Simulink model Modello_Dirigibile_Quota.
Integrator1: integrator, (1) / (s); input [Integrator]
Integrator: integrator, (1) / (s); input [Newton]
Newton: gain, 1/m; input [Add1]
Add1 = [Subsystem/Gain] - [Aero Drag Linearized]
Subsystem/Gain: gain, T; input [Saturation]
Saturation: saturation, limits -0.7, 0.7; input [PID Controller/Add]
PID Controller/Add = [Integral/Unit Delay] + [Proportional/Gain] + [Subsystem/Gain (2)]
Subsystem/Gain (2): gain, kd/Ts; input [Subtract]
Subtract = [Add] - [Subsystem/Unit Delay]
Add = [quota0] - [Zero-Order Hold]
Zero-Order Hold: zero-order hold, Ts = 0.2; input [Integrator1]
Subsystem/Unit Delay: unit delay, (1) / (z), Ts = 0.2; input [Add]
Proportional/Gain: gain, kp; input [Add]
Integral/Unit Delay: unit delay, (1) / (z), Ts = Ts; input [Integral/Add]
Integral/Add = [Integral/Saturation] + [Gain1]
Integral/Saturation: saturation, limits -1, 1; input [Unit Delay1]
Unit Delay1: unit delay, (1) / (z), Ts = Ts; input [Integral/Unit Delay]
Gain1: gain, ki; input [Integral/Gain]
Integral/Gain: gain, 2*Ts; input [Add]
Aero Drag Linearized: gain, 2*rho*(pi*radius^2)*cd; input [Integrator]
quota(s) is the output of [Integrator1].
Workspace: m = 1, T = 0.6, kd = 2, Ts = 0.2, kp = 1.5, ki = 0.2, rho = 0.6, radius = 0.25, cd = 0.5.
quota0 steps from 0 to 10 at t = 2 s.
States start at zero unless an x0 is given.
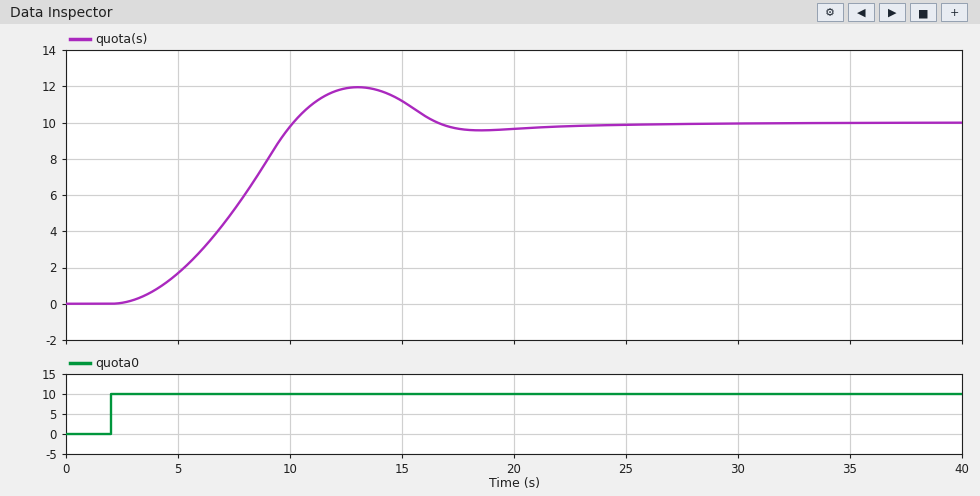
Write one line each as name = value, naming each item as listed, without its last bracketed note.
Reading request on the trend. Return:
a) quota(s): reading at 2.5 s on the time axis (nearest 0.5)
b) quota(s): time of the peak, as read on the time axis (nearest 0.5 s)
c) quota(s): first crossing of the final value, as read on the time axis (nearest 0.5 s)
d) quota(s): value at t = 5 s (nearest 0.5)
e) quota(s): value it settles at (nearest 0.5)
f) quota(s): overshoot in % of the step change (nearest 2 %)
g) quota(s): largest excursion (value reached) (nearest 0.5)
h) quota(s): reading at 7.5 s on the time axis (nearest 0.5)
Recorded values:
quota(s): reading at 2.5 s on the time axis = 0.0
quota(s): time of the peak, as read on the time axis = 13.0 s
quota(s): first crossing of the final value, as read on the time axis = 10.0 s
quota(s): value at t = 5 s = 1.5
quota(s): value it settles at = 10.0
quota(s): overshoot in % of the step change = 20 %
quota(s): largest excursion (value reached) = 12.0
quota(s): reading at 7.5 s on the time axis = 5.0
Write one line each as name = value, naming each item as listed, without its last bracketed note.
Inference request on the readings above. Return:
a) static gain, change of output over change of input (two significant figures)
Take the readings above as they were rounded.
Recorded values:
static gain, change of output over change of input = 1.0
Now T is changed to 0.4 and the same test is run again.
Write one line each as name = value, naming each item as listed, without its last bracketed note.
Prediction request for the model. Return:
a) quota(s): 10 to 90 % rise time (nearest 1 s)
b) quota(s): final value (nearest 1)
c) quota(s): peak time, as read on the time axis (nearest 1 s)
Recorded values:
quota(s): 10 to 90 % rise time = 7 s
quota(s): final value = 10
quota(s): peak time, as read on the time axis = 16 s
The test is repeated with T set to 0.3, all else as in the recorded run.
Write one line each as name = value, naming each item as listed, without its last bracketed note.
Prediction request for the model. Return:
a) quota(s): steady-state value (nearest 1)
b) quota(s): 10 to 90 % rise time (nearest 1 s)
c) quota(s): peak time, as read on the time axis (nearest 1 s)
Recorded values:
quota(s): steady-state value = 10
quota(s): 10 to 90 % rise time = 8 s
quota(s): peak time, as read on the time axis = 18 s
